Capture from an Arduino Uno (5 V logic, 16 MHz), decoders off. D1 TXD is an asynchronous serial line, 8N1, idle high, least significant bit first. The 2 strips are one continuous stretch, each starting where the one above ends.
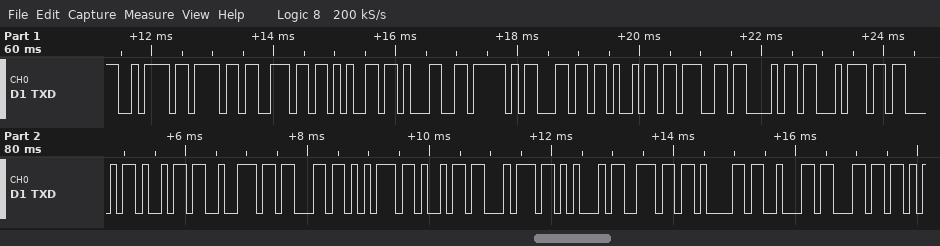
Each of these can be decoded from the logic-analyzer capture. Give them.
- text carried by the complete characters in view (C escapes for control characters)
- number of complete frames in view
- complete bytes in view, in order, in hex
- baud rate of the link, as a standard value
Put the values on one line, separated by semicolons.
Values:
"zone1_lightCircuitEnabl"; 23; 7A 6F 6E 65 31 5F 6C 69 67 68 74 43 69 72 63 75 69 74 45 6E 61 62 6C; 9600 baud
